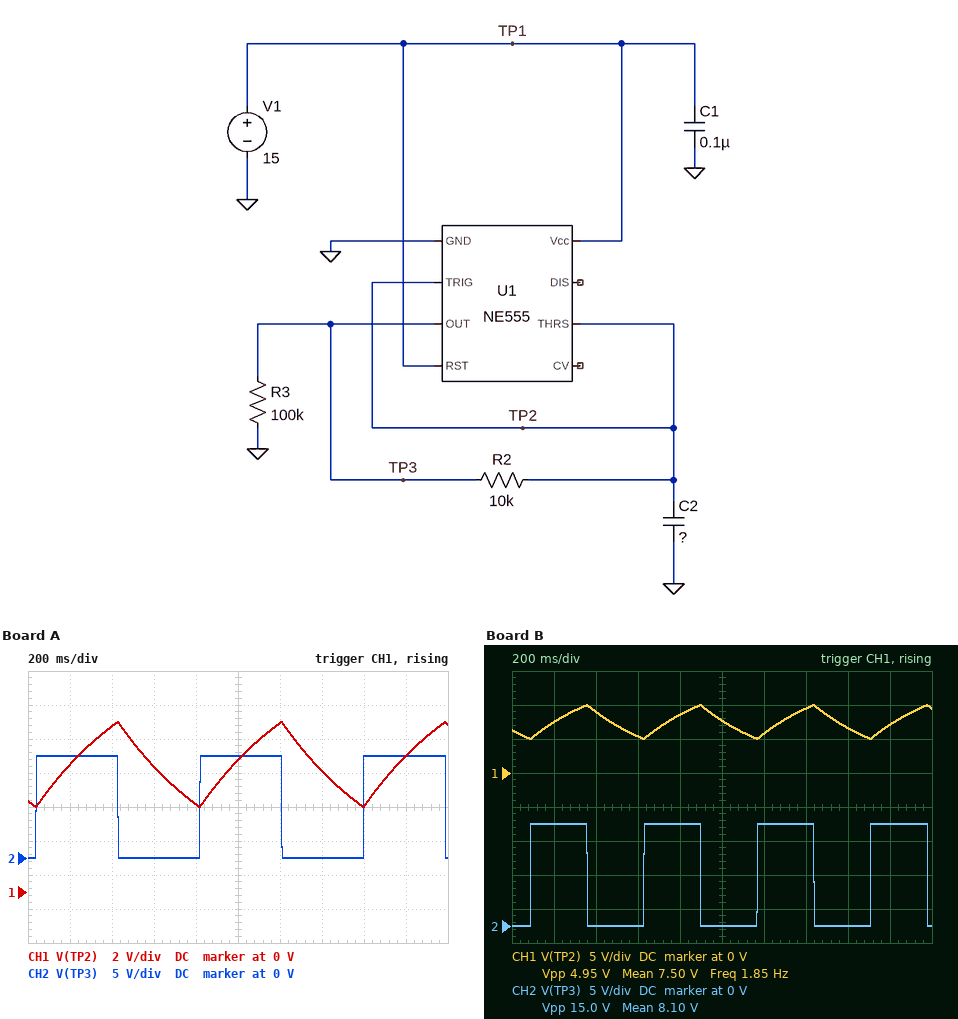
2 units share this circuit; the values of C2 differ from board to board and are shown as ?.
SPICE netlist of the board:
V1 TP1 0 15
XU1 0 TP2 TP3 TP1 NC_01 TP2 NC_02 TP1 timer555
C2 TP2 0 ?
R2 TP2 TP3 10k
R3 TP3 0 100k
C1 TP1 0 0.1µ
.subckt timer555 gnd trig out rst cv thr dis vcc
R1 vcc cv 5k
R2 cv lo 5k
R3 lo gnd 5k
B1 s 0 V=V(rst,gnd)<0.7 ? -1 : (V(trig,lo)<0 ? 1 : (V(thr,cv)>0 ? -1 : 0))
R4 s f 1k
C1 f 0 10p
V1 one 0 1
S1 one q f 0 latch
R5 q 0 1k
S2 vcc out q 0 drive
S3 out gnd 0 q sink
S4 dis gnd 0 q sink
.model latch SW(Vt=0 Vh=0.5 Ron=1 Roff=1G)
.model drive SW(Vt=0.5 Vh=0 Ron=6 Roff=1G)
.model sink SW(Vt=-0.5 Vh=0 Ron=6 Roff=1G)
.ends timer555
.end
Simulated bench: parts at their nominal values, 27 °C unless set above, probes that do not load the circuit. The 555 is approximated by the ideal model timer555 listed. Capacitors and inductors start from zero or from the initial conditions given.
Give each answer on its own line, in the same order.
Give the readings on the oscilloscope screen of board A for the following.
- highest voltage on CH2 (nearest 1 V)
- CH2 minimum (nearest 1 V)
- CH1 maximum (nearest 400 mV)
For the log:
15 V
0 V
10.0 V
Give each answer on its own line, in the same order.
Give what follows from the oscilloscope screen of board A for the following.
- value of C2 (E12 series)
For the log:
56 µF
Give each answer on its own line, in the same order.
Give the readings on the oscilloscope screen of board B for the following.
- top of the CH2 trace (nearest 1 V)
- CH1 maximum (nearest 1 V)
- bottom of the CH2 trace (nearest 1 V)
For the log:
15 V
10 V
0 V
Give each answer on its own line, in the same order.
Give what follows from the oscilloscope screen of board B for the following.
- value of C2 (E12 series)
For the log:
39 µF
